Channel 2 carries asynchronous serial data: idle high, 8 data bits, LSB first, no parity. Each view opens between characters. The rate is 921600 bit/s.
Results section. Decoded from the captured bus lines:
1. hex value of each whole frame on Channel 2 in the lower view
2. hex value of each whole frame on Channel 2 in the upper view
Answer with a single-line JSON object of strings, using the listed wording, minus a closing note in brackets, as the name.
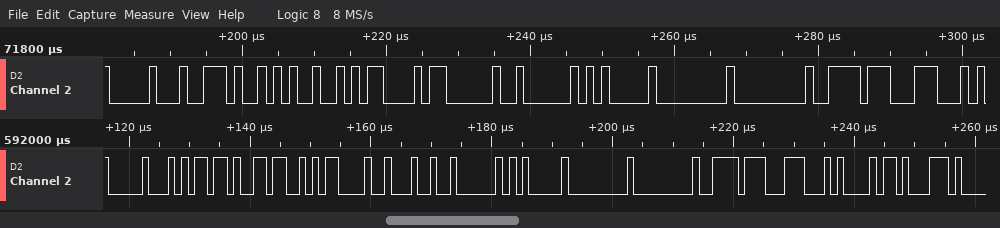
{"hex value of each whole frame on Channel 2 in the lower view": "10, 6D, 36, 0D, 22, 02, 05, 00, 00, DE, 1C, A1, 71", "hex value of each whole frame on Channel 2 in the upper view": "10, 2E, 25, 0D, 03, 02, 05, 00, 00, DE, 1C"}
